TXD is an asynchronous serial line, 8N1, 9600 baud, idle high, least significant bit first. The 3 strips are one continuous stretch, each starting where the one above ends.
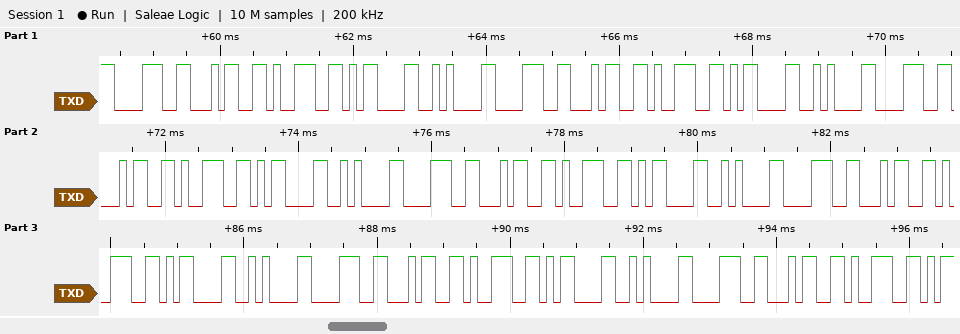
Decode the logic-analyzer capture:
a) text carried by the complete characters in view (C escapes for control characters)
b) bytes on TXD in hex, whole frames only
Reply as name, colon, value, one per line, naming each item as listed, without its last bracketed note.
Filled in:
text carried by the complete characters in view: "849\r\n849\r\n849\r\n849\r\n849\r\n849\r\n849"
bytes on TXD in hex, whole frames only: 38 34 39 0D 0A 38 34 39 0D 0A 38 34 39 0D 0A 38 34 39 0D 0A 38 34 39 0D 0A 38 34 39 0D 0A 38 34 39
